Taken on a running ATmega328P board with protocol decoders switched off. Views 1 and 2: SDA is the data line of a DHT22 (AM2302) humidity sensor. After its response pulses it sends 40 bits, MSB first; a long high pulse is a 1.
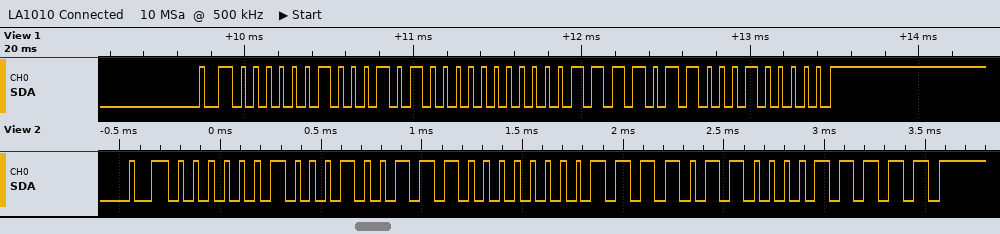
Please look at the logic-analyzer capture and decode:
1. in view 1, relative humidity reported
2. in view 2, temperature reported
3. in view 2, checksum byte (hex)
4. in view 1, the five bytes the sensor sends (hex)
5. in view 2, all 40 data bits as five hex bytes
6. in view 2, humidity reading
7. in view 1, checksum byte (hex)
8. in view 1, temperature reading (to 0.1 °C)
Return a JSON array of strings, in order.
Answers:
["55.2 %", "24.6 °C", "0x1F", "02 28 00 F6 20", "02 27 00 F6 1F", "55.1 %", "0x20", "24.6 °C"]
